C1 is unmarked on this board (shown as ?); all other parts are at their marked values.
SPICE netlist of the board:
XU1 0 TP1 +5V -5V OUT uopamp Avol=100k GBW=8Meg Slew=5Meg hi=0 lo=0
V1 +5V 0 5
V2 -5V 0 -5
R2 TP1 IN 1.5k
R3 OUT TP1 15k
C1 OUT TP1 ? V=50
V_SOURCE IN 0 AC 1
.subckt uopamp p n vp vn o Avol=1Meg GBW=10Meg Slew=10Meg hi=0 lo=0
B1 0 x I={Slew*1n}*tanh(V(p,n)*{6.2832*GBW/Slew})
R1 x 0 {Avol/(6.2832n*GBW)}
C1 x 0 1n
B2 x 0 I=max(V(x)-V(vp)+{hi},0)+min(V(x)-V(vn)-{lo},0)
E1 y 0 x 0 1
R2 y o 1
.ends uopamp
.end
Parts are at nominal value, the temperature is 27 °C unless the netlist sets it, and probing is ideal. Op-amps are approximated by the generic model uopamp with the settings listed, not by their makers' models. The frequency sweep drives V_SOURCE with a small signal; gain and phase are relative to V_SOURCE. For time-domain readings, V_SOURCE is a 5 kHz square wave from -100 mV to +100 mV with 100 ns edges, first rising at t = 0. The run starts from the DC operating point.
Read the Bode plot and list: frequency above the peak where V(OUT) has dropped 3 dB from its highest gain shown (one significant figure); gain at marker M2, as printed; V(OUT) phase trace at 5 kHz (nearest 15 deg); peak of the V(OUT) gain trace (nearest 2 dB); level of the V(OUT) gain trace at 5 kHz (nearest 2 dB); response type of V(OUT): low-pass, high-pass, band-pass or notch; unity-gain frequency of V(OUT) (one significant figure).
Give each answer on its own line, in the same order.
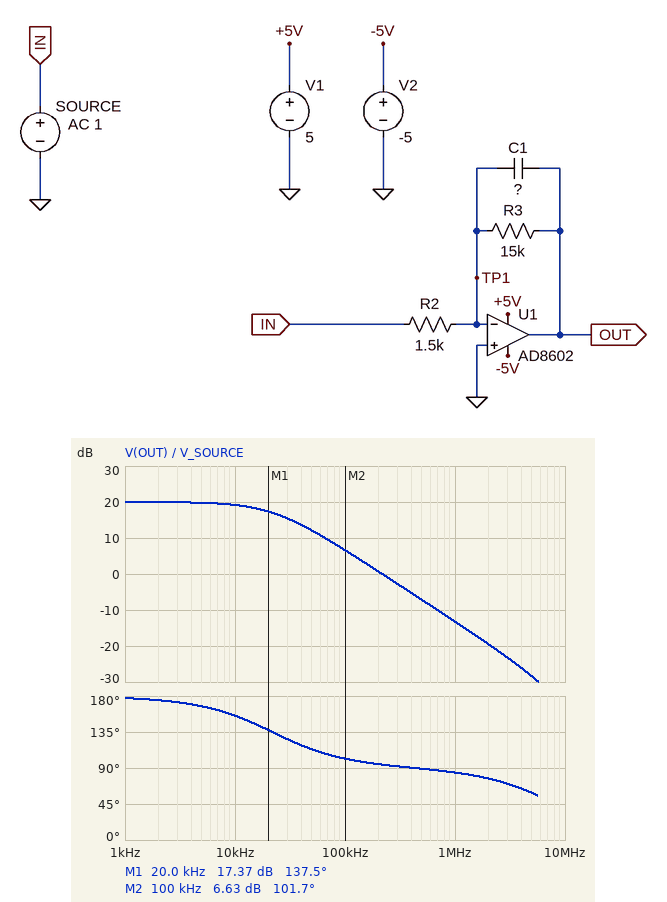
20 kHz
6.63 dB
165 deg
20 dB
20 dB
low-pass
200 kHz
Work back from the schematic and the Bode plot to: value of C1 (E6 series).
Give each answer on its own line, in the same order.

470 pF
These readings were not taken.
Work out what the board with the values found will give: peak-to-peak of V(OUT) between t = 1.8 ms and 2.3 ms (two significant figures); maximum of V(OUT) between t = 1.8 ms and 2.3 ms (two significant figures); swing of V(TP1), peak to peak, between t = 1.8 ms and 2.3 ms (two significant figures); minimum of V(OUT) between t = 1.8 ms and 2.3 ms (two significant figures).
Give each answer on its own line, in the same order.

2.0 V
1.0 V
11 mV
-1.0 V
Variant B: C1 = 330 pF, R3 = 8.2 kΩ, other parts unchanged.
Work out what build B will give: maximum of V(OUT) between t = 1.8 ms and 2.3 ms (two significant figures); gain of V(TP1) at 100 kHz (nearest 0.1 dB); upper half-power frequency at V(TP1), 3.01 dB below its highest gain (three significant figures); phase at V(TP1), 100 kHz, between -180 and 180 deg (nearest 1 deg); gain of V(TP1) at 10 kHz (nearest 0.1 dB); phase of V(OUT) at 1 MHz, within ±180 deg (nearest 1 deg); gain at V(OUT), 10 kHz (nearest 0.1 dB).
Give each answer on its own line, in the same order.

550 mV
-29.5 dB
8.43 MHz
29 deg
-43.4 dB
86 deg
14.6 dB
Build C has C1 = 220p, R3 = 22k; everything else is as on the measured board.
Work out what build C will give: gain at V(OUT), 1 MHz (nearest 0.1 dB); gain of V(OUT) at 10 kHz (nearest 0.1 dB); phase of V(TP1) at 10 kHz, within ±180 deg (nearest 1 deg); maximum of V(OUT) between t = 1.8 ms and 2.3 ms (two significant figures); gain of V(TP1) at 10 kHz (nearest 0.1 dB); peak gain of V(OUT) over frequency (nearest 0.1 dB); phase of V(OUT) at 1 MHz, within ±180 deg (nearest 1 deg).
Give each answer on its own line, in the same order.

-6.9 dB
22.9 dB
72 deg
1.5 V
-35.2 dB
23.3 dB
85 deg
